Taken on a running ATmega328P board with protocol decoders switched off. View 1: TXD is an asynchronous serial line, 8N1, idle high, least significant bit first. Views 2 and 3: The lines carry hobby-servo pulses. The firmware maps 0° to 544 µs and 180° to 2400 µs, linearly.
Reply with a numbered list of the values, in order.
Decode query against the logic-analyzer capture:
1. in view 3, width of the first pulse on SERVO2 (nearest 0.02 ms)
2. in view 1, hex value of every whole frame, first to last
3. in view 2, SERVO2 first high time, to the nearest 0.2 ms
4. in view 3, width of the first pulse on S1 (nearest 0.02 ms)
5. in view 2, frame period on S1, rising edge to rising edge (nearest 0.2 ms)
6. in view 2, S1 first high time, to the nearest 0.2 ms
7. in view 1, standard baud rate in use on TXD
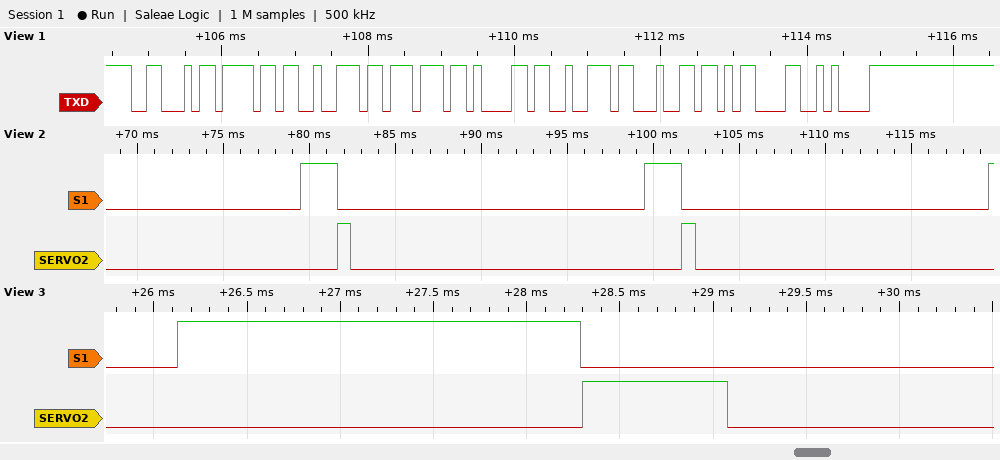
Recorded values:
1. 0.78 ms
2. 46 6F 72 77 61 72 64 0D 0A
3. 0.8 ms
4. 2.16 ms
5. 20.0 ms
6. 2.2 ms
7. 9600 baud
